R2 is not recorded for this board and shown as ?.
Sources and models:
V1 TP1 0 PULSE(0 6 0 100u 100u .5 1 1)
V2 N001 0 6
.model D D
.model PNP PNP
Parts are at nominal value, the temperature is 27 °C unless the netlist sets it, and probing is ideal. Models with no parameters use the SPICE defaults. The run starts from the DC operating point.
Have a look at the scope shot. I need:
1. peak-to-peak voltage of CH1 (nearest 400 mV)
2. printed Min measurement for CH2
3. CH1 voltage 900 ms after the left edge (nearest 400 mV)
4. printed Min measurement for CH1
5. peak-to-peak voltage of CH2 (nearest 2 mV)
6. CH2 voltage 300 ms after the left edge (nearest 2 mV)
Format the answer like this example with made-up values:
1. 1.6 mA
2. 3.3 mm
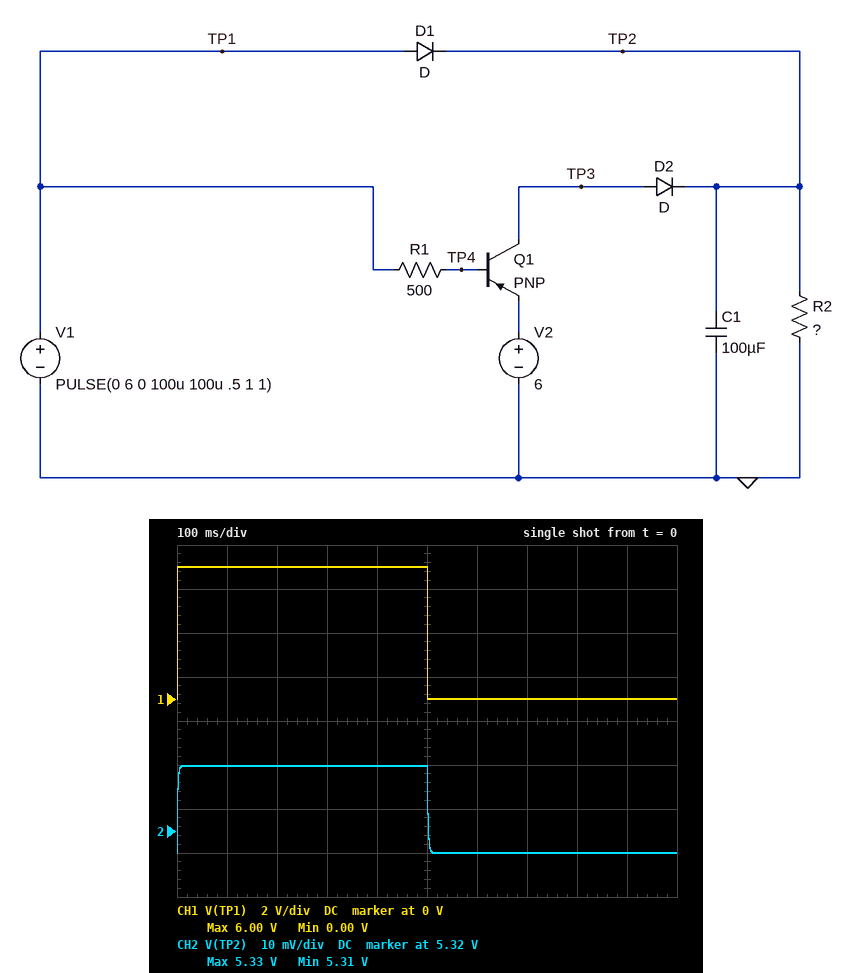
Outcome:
1. 6.0 V
2. 5.31 V
3. 0 V
4. 0.00 V
5. 20 mV
6. 5.334 V
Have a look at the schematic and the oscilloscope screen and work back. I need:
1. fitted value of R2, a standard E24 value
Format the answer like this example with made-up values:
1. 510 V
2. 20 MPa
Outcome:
1. 3.6 kΩ
